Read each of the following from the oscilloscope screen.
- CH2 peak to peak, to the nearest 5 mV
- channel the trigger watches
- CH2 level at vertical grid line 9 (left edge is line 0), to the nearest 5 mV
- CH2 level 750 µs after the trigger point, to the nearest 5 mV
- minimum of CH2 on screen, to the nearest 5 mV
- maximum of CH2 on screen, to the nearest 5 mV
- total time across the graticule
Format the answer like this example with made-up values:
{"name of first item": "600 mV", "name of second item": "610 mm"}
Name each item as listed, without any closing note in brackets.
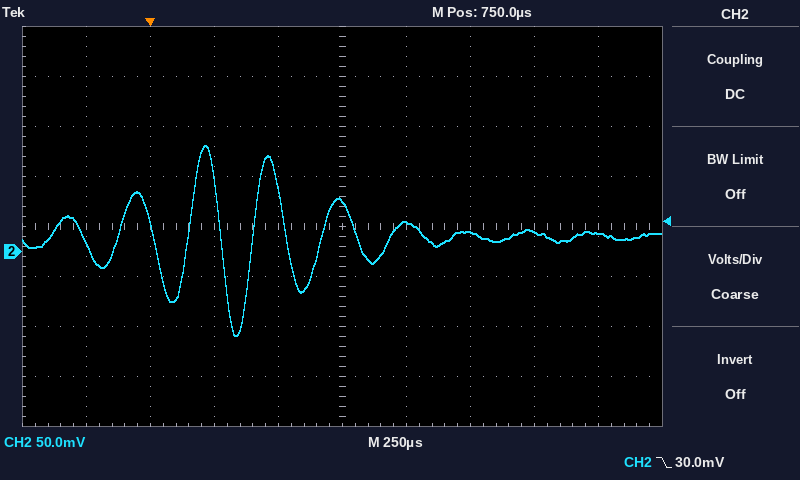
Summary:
{"CH2 peak to peak, to the nearest 5 mV": "190 mV", "channel the trigger watches": "CH2", "CH2 level at vertical grid line 9 (left edge is line 0), to the nearest 5 mV": "20 mV", "CH2 level 750 µs after the trigger point, to the nearest 5 mV": "50 mV", "minimum of CH2 on screen, to the nearest 5 mV": "-85 mV", "maximum of CH2 on screen, to the nearest 5 mV": "105 mV", "total time across the graticule": "2.5 ms"}
